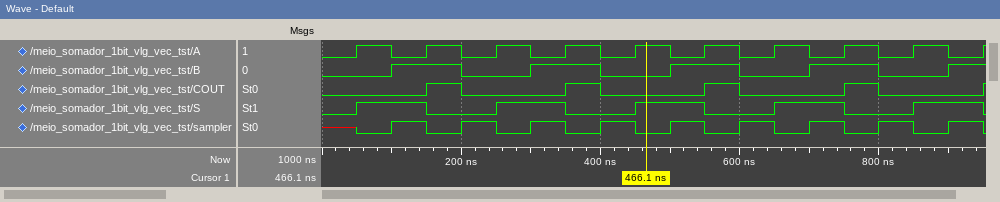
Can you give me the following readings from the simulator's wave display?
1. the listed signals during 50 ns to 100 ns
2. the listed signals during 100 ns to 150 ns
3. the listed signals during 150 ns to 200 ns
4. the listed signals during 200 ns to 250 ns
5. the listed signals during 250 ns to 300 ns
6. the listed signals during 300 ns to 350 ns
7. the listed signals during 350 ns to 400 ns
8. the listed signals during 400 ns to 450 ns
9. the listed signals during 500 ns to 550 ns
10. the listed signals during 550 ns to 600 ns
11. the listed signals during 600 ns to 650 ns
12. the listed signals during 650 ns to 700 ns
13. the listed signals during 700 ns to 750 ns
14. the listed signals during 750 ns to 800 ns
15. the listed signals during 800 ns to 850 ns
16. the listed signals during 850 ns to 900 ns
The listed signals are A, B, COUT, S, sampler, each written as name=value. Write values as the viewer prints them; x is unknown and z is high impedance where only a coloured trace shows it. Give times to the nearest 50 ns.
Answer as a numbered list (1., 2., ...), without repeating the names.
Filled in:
1. A=1, B=0, COUT=0, S=1, sampler=0
2. A=0, B=1, COUT=0, S=1, sampler=1
3. A=1, B=1, COUT=1, S=0, sampler=0
4. A=0, B=0, COUT=0, S=0, sampler=1
5. A=1, B=0, COUT=0, S=1, sampler=0
6. A=0, B=1, COUT=0, S=1, sampler=1
7. A=1, B=1, COUT=1, S=0, sampler=0
8. A=0, B=0, COUT=0, S=0, sampler=1
9. A=0, B=1, COUT=0, S=1, sampler=1
10. A=1, B=1, COUT=1, S=0, sampler=0
11. A=0, B=0, COUT=0, S=0, sampler=1
12. A=1, B=0, COUT=0, S=1, sampler=0
13. A=0, B=1, COUT=0, S=1, sampler=1
14. A=1, B=1, COUT=1, S=0, sampler=0
15. A=0, B=0, COUT=0, S=0, sampler=1
16. A=1, B=0, COUT=0, S=1, sampler=0
